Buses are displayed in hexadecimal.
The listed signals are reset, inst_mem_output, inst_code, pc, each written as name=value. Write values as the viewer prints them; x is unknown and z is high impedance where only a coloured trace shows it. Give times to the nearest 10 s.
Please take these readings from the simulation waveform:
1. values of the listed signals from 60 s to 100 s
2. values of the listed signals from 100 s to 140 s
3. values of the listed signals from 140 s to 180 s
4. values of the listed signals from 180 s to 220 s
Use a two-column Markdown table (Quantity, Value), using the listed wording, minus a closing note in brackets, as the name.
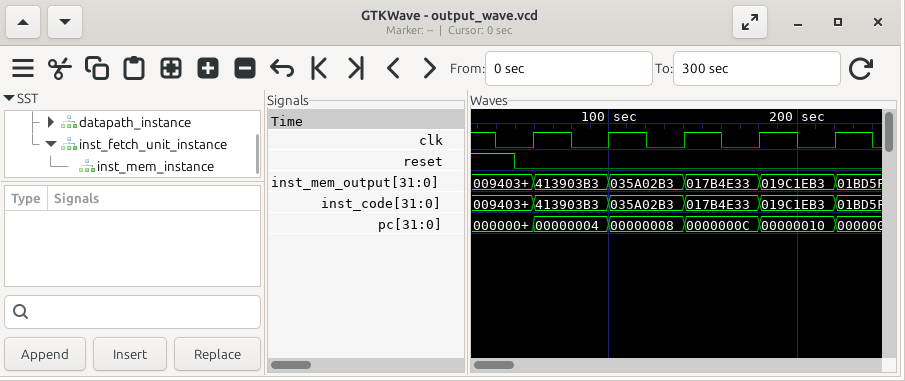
| Quantity | Value |
|---|---|
| values of the listed signals from 60 s to 100 s | reset=0, inst_mem_output=413903B3, inst_code=413903B3, pc=00000004 |
| values of the listed signals from 100 s to 140 s | reset=0, inst_mem_output=035A02B3, inst_code=035A02B3, pc=00000008 |
| values of the listed signals from 140 s to 180 s | reset=0, inst_mem_output=017B4E33, inst_code=017B4E33, pc=0000000C |
| values of the listed signals from 180 s to 220 s | reset=0, inst_mem_output=019C1EB3, inst_code=019C1EB3, pc=00000010 |
